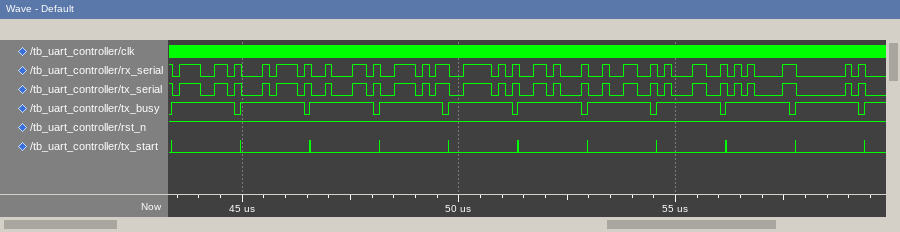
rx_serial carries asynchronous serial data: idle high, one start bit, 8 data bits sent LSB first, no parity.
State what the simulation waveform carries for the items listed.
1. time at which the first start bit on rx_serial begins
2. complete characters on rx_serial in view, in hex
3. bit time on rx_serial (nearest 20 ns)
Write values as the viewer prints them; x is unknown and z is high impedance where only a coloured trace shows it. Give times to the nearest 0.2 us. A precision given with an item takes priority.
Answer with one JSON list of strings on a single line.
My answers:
["43.4 us", "67, 74, 62, AE, 5E, 16, 32, 31, 85, 40", "160 ns"]
